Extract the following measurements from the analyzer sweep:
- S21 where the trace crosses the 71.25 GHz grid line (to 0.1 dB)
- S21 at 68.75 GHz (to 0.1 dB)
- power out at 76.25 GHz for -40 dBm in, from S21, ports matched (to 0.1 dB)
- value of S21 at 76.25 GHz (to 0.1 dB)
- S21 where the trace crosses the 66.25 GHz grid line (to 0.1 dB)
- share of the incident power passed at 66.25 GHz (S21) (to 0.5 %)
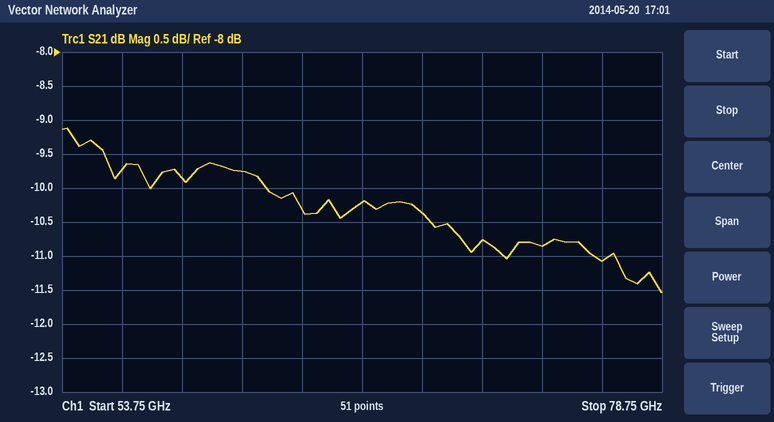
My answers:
-10.8 dB
-10.4 dB
-51.1 dBm
-11.1 dB
-10.2 dB
9.5 %
